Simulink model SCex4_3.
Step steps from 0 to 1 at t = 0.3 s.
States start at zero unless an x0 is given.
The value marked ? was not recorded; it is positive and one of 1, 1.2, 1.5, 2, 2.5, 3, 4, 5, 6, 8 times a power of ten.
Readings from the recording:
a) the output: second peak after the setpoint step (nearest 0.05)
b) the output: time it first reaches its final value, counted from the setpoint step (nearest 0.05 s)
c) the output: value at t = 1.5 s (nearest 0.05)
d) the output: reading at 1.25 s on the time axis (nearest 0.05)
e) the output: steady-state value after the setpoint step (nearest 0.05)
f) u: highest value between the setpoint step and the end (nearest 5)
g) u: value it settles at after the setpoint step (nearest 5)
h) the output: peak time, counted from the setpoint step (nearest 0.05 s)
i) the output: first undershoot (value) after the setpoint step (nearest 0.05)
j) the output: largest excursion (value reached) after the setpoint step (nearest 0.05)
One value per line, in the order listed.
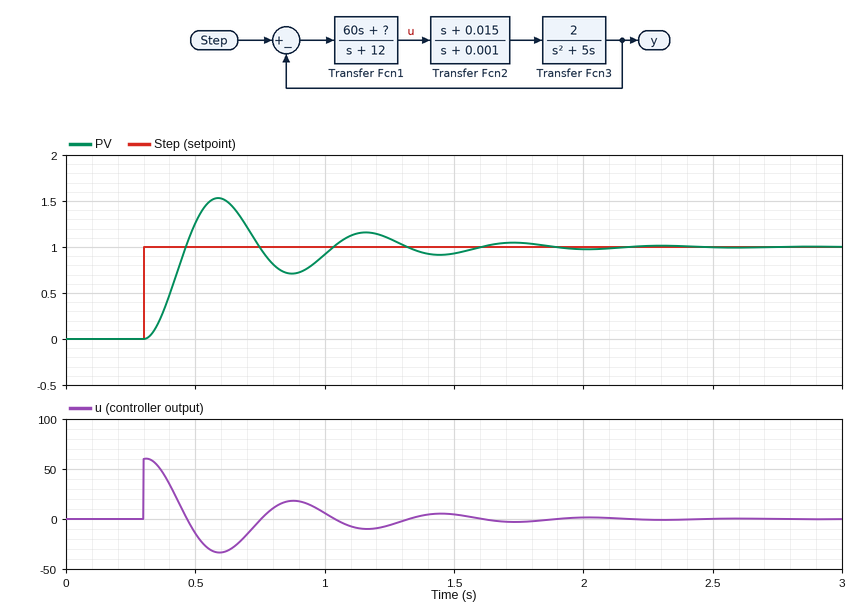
1.15
0.15 s
0.95
1.10
1.00
60
0
0.30 s
0.70
1.55
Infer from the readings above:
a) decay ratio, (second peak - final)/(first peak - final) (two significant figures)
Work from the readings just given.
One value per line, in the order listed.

0.27
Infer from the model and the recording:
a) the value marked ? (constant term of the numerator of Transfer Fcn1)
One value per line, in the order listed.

800
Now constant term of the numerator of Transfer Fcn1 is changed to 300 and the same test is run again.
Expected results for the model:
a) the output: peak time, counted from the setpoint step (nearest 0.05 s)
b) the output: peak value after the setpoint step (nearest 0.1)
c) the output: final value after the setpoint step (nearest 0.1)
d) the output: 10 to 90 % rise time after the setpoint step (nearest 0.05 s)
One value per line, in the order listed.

0.35 s
1.1
1.0
0.15 s
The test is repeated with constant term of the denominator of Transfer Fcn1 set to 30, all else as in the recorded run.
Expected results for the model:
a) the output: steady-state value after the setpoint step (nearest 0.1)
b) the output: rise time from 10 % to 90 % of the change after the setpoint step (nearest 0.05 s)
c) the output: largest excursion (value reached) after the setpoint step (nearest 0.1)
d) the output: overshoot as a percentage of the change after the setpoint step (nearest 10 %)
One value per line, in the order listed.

1.0
0.20 s
1.2
20 %
